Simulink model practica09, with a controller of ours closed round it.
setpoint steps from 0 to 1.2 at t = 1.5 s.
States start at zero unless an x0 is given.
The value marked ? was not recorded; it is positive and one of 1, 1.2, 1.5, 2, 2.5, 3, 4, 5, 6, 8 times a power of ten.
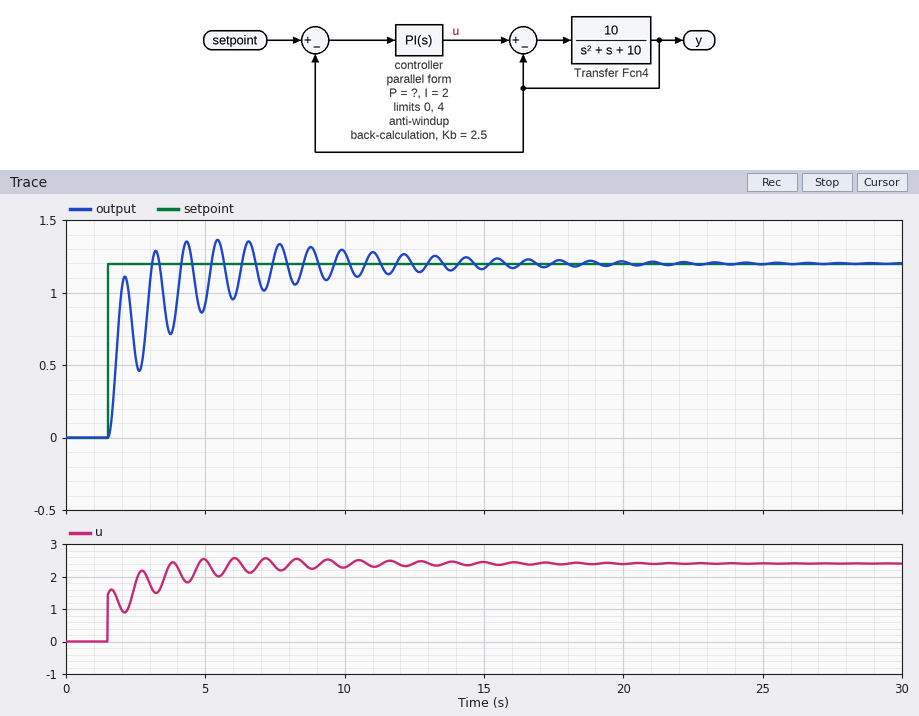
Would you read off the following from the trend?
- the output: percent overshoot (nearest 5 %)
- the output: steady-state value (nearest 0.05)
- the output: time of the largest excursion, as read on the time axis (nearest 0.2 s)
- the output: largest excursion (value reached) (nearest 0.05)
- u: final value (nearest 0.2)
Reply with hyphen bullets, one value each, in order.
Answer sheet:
- 15 %
- 1.20
- 5.4 s
- 1.35
- 2.4
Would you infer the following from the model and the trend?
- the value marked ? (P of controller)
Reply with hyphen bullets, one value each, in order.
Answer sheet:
- 1.2
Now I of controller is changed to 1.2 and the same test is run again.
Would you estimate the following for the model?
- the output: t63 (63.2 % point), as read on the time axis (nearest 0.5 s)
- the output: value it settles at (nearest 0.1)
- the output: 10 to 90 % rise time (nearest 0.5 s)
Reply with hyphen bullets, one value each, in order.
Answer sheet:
- 2.0 s
- 1.2
- 2.5 s
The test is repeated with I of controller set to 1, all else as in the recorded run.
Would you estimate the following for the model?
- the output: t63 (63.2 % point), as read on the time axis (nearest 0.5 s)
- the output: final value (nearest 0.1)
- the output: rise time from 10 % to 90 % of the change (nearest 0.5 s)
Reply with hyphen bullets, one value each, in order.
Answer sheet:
- 2.0 s
- 1.2
- 3.5 s
